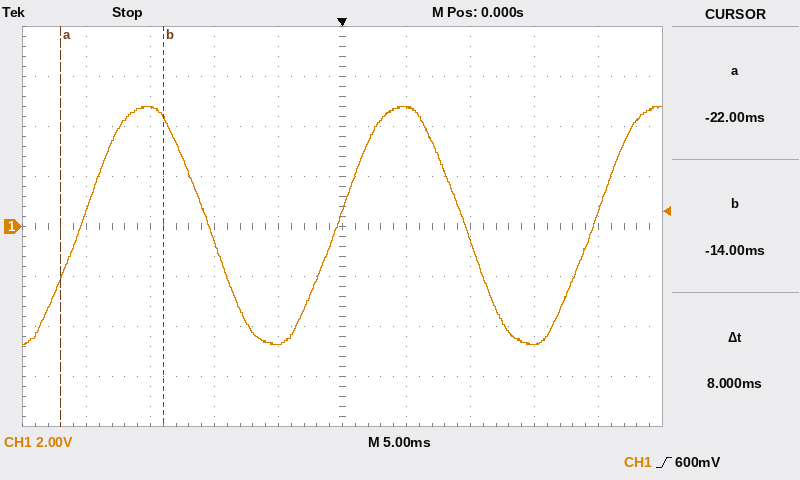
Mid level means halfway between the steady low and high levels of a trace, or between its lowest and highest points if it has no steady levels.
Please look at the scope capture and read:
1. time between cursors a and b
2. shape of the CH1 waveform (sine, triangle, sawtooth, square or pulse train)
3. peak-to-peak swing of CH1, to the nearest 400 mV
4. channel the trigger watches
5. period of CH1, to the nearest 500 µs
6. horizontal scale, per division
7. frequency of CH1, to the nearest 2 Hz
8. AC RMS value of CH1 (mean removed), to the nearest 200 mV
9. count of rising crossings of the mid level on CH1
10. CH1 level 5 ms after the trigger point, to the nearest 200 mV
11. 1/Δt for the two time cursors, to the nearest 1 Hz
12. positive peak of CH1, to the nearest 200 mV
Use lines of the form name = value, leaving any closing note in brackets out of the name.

time between cursors a and b = 8 ms
shape of the CH1 waveform = sine
peak-to-peak swing of CH1, to the nearest 400 mV = 9.6 V
channel the trigger watches = CH1
period of CH1, to the nearest 500 µs = 20.0 ms
horizontal scale, per division = 5 ms
frequency of CH1, to the nearest 2 Hz = 50 Hz
AC RMS value of CH1 (mean removed), to the nearest 200 mV = 3.4 V
count of rising crossings of the mid level on CH1 = 3
CH1 level 5 ms after the trigger point, to the nearest 200 mV = 4.8 V
1/Δt for the two time cursors, to the nearest 1 Hz = 125 Hz
positive peak of CH1, to the nearest 200 mV = 4.8 V
